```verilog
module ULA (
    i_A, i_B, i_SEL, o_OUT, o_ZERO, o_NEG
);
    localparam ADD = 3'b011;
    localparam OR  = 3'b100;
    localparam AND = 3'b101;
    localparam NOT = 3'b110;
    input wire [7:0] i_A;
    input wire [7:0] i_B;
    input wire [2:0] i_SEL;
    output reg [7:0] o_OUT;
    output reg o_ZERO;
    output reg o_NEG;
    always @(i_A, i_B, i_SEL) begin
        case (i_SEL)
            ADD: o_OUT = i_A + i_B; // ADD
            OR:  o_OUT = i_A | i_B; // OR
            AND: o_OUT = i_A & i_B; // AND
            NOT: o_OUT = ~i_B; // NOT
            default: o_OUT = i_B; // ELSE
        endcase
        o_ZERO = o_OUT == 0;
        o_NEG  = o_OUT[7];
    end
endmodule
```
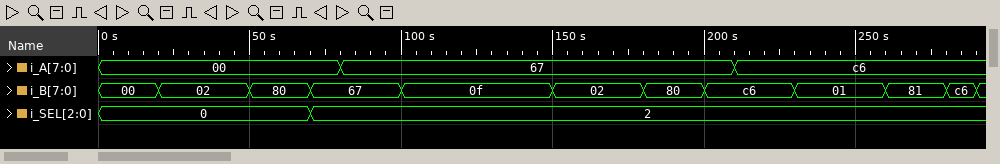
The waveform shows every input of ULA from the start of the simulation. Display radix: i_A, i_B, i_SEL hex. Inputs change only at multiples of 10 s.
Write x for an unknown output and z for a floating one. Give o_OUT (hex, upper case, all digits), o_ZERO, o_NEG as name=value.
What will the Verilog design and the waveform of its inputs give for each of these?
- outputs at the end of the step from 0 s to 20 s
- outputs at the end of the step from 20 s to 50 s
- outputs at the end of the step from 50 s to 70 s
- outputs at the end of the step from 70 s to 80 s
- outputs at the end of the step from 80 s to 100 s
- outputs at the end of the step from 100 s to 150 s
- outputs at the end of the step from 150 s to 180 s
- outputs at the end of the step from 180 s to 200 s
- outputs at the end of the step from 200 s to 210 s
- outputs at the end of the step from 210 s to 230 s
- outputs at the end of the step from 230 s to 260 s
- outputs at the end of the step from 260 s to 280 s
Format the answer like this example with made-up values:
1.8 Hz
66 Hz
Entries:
o_OUT=00, o_ZERO=1, o_NEG=0
o_OUT=02, o_ZERO=0, o_NEG=0
o_OUT=80, o_ZERO=0, o_NEG=1
o_OUT=67, o_ZERO=0, o_NEG=0
o_OUT=67, o_ZERO=0, o_NEG=0
o_OUT=0F, o_ZERO=0, o_NEG=0
o_OUT=02, o_ZERO=0, o_NEG=0
o_OUT=80, o_ZERO=0, o_NEG=1
o_OUT=C6, o_ZERO=0, o_NEG=1
o_OUT=C6, o_ZERO=0, o_NEG=1
o_OUT=01, o_ZERO=0, o_NEG=0
o_OUT=81, o_ZERO=0, o_NEG=1
